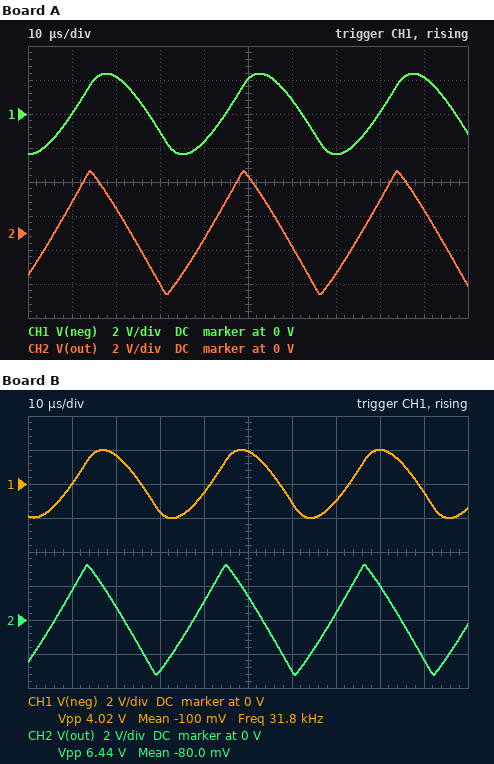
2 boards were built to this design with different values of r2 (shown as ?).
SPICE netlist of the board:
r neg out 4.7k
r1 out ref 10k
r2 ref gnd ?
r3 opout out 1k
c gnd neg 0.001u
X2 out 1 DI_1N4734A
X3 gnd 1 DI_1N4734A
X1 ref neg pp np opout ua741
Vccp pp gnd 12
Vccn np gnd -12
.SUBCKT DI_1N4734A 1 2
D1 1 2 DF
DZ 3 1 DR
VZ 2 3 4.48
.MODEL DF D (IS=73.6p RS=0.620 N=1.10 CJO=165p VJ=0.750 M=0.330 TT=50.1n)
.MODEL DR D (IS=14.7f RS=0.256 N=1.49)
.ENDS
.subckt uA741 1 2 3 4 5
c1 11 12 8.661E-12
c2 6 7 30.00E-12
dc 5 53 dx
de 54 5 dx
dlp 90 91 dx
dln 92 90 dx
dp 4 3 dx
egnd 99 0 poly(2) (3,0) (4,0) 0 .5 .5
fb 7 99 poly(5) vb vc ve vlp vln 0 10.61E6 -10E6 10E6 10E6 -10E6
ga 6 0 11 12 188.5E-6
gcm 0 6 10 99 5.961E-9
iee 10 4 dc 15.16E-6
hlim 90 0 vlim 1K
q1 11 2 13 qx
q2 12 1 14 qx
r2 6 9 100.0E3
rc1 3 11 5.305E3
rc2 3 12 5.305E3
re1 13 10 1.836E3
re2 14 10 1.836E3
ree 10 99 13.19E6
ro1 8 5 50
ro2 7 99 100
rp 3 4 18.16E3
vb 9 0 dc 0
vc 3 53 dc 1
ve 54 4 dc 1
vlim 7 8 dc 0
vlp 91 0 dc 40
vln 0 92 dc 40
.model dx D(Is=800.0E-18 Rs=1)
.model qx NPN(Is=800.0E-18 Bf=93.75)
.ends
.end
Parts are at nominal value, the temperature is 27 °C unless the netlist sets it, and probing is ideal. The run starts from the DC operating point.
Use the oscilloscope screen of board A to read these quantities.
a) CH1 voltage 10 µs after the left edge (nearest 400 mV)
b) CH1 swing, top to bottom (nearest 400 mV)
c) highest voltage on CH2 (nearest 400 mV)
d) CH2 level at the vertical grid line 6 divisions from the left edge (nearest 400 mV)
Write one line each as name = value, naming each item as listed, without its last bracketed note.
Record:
CH1 voltage 10 µs after the left edge = 0 V
CH1 swing, top to bottom = 4.8 V
highest voltage on CH2 = 3.6 V
CH2 level at the vertical grid line 6 divisions from the left edge = -800 mV
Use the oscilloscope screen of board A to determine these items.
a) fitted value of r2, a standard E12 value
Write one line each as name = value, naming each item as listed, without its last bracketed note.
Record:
fitted value of r2, a standard E12 value = 8.2 kΩ
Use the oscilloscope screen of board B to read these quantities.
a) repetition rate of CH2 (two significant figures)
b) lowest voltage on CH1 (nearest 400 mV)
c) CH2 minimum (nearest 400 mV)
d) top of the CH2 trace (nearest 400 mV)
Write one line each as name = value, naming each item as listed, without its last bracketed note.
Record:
repetition rate of CH2 = 32 kHz
lowest voltage on CH1 = -2.0 V
CH2 minimum = -3.2 V
top of the CH2 trace = 3.2 V
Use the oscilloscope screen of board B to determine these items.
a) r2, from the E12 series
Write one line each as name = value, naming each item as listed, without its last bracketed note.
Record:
r2, from the E12 series = 6.8 kΩ
